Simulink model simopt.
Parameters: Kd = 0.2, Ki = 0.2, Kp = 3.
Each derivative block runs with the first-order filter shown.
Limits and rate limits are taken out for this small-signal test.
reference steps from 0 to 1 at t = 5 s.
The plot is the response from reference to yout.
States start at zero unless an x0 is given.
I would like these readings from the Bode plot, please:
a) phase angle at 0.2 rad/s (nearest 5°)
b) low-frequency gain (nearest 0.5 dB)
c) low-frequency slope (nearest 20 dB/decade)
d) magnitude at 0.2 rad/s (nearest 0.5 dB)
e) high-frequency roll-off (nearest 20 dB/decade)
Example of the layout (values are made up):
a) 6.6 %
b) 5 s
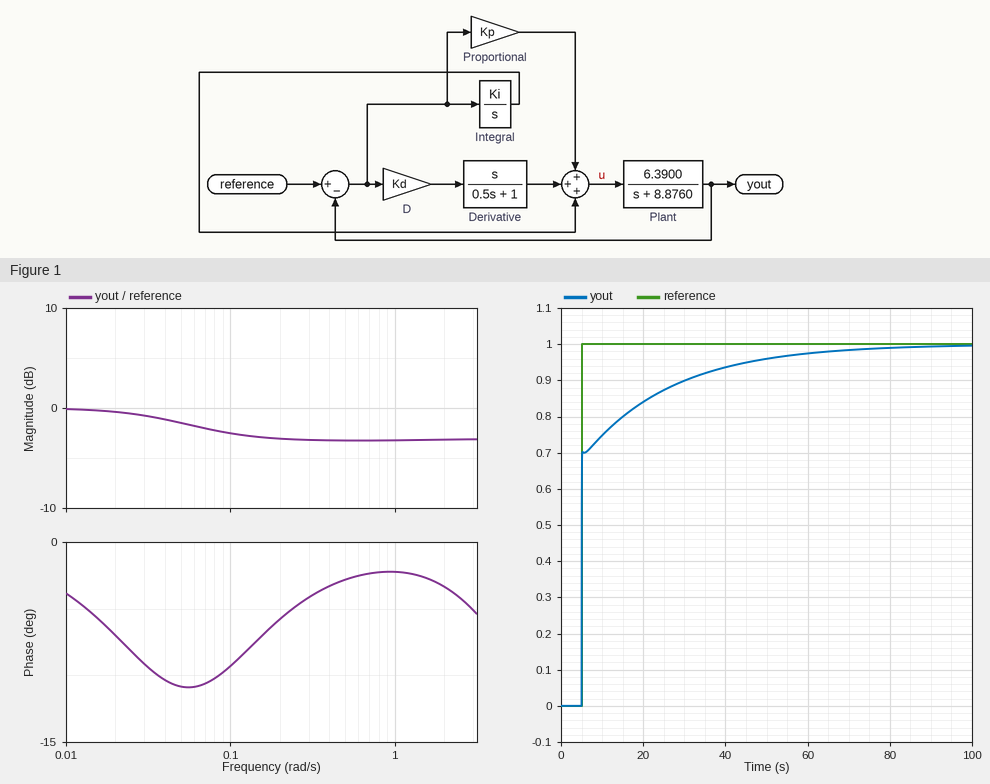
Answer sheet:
a) -5°
b) 0.0 dB
c) 0 dB/decade
d) -3.0 dB
e) 0 dB/decade
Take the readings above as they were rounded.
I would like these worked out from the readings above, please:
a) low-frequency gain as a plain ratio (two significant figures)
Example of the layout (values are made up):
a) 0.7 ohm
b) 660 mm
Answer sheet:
a) 1.0
